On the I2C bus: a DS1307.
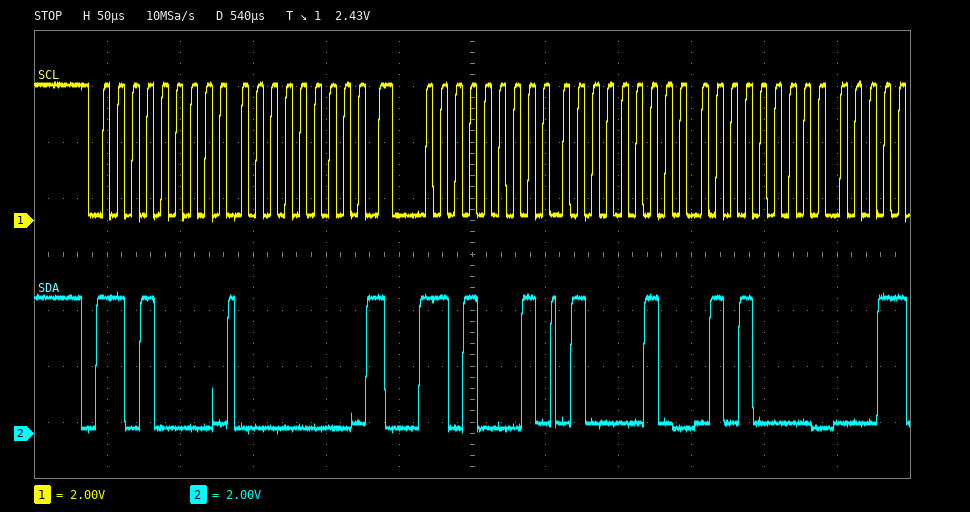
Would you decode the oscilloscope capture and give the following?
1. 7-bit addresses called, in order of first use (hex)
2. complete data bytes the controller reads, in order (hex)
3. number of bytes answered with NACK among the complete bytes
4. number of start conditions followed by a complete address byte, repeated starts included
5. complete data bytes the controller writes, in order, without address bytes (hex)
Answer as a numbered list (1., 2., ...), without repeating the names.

1. 0x68
2. 42 50
3. 0
4. 2
5. 00
